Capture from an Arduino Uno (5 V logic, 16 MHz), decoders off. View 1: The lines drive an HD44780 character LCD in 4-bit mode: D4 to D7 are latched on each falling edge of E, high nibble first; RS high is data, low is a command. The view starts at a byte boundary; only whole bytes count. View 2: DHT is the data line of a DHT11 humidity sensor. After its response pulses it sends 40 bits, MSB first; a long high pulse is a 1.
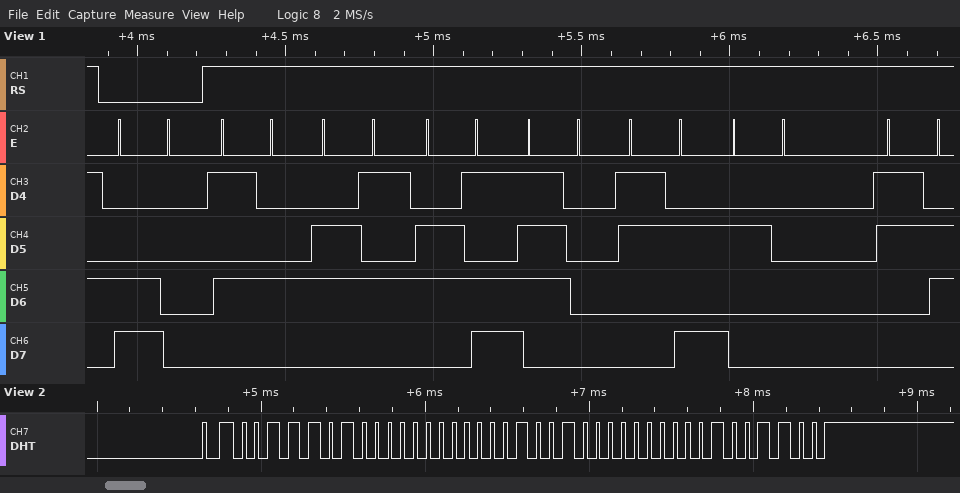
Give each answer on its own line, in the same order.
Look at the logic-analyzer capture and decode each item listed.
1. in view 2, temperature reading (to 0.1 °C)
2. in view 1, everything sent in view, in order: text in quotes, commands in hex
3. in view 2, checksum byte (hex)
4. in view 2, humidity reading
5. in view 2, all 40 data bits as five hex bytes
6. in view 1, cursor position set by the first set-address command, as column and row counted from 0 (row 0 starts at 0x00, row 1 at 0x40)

18.0 °C
0xC0 "Temp: 6"
0x4C
58 %
3A 00 12 00 4C
column 0, row 1
